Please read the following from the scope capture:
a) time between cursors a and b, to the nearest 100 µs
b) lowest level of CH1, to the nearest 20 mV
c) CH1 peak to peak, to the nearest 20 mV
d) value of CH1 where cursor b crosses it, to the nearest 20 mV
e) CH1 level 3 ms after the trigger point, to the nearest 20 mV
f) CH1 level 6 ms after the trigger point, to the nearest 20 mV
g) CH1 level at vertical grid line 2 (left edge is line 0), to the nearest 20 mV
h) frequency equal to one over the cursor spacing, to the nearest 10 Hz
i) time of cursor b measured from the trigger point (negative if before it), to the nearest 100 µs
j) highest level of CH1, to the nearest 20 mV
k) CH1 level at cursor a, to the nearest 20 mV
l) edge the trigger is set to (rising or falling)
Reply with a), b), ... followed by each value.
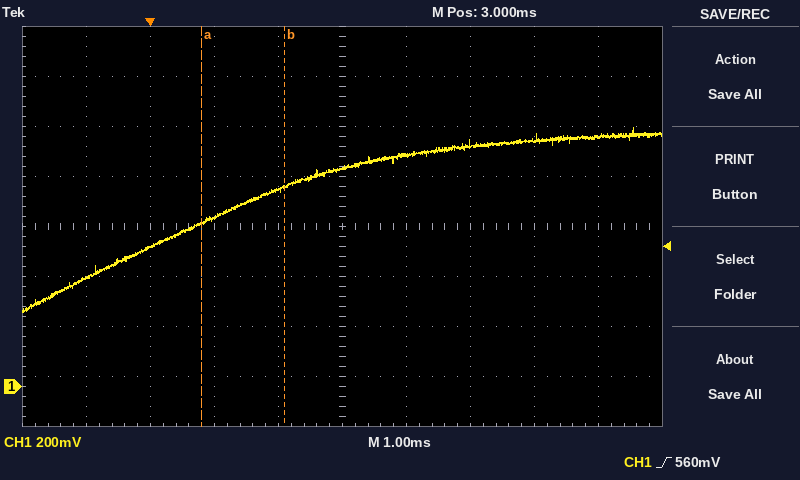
a) 1.3 ms
b) 300 mV
c) 740 mV
d) 800 mV
e) 880 mV
f) 1.00 V
g) 560 mV
h) 770 Hz
i) +2.1 ms
j) 1.04 V
k) 660 mV
l) rising
